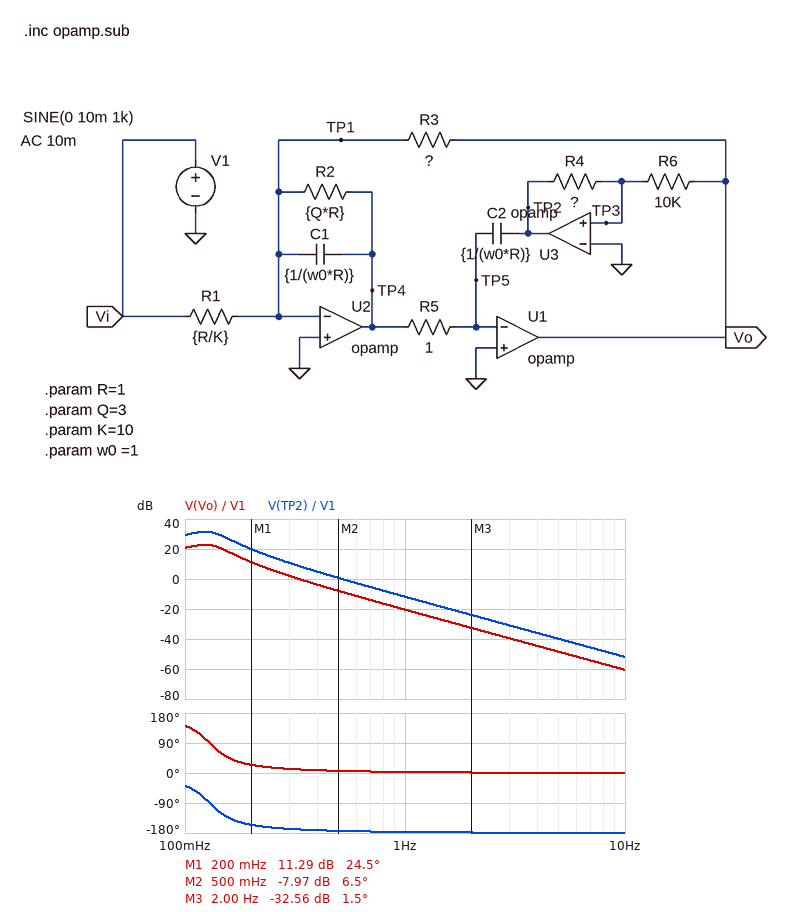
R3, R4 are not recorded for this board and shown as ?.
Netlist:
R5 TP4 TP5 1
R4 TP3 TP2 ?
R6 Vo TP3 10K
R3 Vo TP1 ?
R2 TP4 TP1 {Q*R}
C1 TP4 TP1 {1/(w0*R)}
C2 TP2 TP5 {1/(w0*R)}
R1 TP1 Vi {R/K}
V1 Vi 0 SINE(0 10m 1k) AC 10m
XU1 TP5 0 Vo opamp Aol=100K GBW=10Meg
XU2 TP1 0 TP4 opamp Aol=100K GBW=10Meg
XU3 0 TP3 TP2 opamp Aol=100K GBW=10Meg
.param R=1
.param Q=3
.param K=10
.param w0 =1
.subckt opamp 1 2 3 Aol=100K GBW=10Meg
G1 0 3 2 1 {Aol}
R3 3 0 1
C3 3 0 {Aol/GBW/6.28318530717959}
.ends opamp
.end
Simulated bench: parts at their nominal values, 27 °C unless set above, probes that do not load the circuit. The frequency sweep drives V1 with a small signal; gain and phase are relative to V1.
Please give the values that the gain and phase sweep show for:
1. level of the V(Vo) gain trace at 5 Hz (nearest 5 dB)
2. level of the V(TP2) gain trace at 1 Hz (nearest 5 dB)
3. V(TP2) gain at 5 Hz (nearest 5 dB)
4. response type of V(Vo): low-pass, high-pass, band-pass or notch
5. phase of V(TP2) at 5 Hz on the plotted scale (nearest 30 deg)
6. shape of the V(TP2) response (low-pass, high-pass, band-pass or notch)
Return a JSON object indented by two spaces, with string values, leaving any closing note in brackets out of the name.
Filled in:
{
  "level of the V(Vo) gain trace at 5 Hz": "-50 dB",
  "level of the V(TP2) gain trace at 1 Hz": "-10 dB",
  "V(TP2) gain at 5 Hz": "-40 dB",
  "response type of V(Vo): low-pass, high-pass, band-pass or notch": "low-pass",
  "phase of V(TP2) at 5 Hz on the plotted scale": "-180 deg",
  "shape of the V(TP2) response": "low-pass"
}
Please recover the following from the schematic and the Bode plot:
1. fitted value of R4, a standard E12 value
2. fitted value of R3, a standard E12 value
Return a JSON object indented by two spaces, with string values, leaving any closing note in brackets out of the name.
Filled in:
{
  "fitted value of R4, a standard E12 value": "27 kΩ",
  "fitted value of R3, a standard E12 value": "0.56 Ω"
}
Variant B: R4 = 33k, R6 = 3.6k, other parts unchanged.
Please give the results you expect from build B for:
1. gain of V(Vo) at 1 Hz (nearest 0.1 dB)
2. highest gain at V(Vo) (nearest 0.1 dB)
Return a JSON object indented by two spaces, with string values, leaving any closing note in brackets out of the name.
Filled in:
{
  "gain of V(Vo) at 1 Hz": "-31.1 dB",
  "highest gain at V(Vo)": "18.1 dB"
}
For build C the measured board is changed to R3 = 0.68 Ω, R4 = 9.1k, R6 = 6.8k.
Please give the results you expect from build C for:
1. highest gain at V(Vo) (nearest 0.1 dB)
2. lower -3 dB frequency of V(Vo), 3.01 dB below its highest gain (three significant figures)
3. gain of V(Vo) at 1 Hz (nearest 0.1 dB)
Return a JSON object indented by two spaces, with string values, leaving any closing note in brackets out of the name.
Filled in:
{
  "highest gain at V(Vo)": "26.7 dB",
  "lower -3 dB frequency of V(Vo), 3.01 dB below its highest gain": "133 mHz",
  "gain of V(Vo) at 1 Hz": "-14.2 dB"
}
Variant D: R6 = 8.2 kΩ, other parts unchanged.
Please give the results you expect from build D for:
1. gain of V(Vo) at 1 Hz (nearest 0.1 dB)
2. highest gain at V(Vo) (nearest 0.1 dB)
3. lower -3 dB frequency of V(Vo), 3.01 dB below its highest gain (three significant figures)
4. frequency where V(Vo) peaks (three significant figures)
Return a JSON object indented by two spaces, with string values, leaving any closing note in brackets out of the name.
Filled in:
{
  "gain of V(Vo) at 1 Hz": "-22.2 dB",
  "highest gain at V(Vo)": "22.1 dB",
  "lower -3 dB frequency of V(Vo), 3.01 dB below its highest gain": "79.2 mHz",
  "frequency where V(Vo) peaks": "111 mHz"
}
